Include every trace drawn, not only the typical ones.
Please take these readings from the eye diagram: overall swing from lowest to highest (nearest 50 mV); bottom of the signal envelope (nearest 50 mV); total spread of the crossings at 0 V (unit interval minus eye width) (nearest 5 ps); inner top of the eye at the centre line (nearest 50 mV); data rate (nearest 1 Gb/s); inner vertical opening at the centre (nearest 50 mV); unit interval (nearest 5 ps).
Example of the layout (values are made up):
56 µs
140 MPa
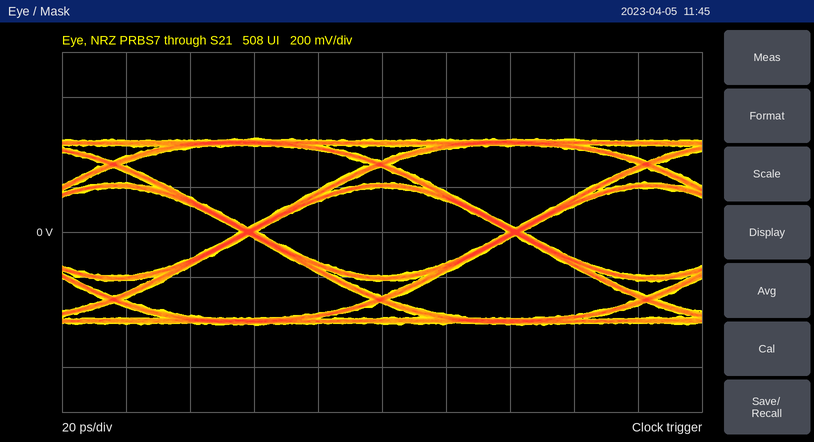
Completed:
850 mV
-400 mV
5 ps
200 mV
12 Gb/s
400 mV
85 ps
